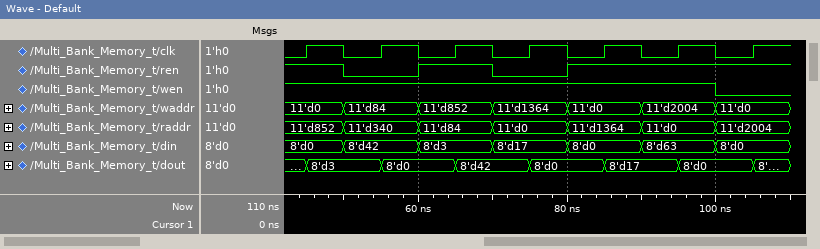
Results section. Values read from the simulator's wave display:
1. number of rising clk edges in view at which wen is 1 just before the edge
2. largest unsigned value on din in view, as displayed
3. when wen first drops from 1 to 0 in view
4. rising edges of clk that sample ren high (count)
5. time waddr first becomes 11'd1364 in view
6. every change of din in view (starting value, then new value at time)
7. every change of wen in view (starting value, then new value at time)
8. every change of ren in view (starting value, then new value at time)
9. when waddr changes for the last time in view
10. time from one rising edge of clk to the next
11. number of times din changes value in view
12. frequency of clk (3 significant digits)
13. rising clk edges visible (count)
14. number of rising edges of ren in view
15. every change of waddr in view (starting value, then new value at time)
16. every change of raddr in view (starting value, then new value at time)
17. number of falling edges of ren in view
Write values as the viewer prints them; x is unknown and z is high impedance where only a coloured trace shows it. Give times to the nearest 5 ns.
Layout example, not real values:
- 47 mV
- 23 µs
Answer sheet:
- 6
- 8'd63
- 100 ns
- 5
- 70 ns
- 8'd0, 8'd42 at 50 ns, 8'd3 at 60 ns, 8'd17 at 70 ns, 8'd0 at 80 ns, 8'd63 at 90 ns, 8'd0 at 100 ns
- 1, 0 at 100 ns
- 1, 0 at 50 ns, 1 at 60 ns, 0 at 70 ns, 1 at 80 ns
- 100 ns
- 10 ns
- 6
- 100 MHz
- 7
- 2
- 11'd0, 11'd84 at 50 ns, 11'd852 at 60 ns, 11'd1364 at 70 ns, 11'd0 at 80 ns, 11'd2004 at 90 ns, 11'd0 at 100 ns
- 11'd852, 11'd340 at 50 ns, 11'd84 at 60 ns, 11'd0 at 70 ns, 11'd1364 at 80 ns, 11'd0 at 90 ns, 11'd2004 at 100 ns
- 2
